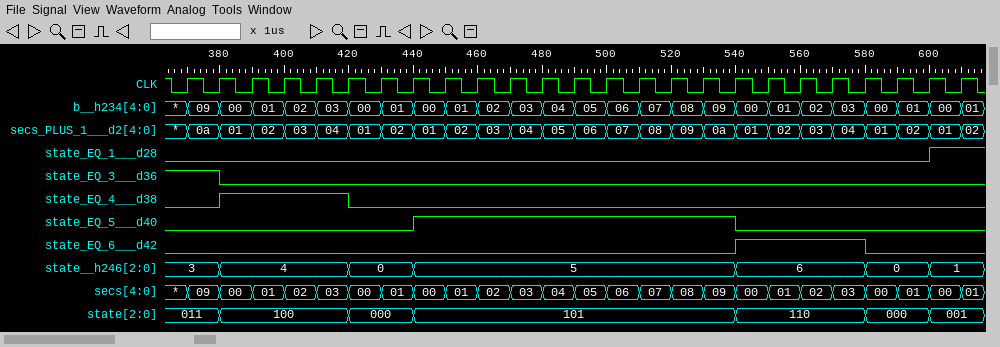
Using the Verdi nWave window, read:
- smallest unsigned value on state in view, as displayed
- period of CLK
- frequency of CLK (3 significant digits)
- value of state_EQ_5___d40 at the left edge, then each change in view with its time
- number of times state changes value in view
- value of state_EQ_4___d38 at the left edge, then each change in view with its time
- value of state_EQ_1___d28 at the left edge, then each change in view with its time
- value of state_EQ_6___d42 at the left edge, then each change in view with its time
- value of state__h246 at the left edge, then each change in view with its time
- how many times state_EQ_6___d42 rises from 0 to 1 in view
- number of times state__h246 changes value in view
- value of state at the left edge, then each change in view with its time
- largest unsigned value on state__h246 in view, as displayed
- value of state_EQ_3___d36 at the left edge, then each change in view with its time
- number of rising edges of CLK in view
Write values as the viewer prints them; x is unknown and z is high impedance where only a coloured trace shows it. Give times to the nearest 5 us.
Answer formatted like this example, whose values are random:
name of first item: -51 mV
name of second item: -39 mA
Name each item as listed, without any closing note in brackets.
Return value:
smallest unsigned value on state in view, as displayed: 000
period of CLK: 10 us
frequency of CLK: 100 kHz
value of state_EQ_5___d40 at the left edge, then each change in view with its time: 0, 1 at 440 us, 0 at 540 us
number of times state changes value in view: 6
value of state_EQ_4___d38 at the left edge, then each change in view with its time: 0, 1 at 380 us, 0 at 420 us
value of state_EQ_1___d28 at the left edge, then each change in view with its time: 0, 1 at 600 us
value of state_EQ_6___d42 at the left edge, then each change in view with its time: 0, 1 at 540 us, 0 at 580 us
value of state__h246 at the left edge, then each change in view with its time: 3, 4 at 380 us, 0 at 420 us, 5 at 440 us, 6 at 540 us, 0 at 580 us, 1 at 600 us
how many times state_EQ_6___d42 rises from 0 to 1 in view: 1
number of times state__h246 changes value in view: 6
value of state at the left edge, then each change in view with its time: 011, 100 at 380 us, 000 at 420 us, 101 at 440 us, 110 at 540 us, 000 at 580 us, 001 at 600 us
largest unsigned value on state__h246 in view, as displayed: 6
value of state_EQ_3___d36 at the left edge, then each change in view with its time: 1, 0 at 380 us
number of rising edges of CLK in view: 25
